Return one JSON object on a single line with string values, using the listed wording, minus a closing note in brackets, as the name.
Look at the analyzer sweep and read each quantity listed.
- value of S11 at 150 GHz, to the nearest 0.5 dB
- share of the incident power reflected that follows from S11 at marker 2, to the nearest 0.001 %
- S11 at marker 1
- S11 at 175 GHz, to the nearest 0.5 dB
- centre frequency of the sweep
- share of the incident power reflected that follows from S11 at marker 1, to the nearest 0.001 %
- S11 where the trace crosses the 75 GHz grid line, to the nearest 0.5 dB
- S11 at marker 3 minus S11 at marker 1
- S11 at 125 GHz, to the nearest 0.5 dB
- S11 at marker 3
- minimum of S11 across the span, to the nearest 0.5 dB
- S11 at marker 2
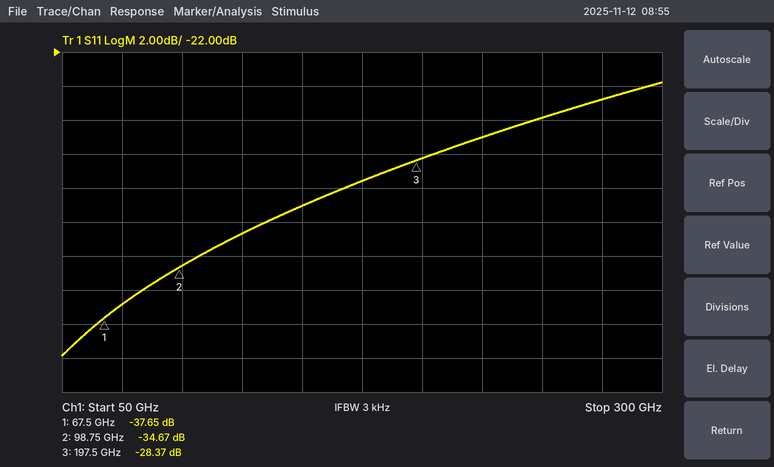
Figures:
{"value of S11 at 150 GHz, to the nearest 0.5 dB": "-31.0 dB", "share of the incident power reflected that follows from S11 at marker 2, to the nearest 0.001 %": "0.034 %", "S11 at marker 1": "-37.65 dB", "S11 at 175 GHz, to the nearest 0.5 dB": "-29.5 dB", "centre frequency of the sweep": "175 GHz", "share of the incident power reflected that follows from S11 at marker 1, to the nearest 0.001 %": "0.017 %", "S11 where the trace crosses the 75 GHz grid line, to the nearest 0.5 dB": "-37.0 dB", "S11 at marker 3 minus S11 at marker 1": "9.28 dB", "S11 at 125 GHz, to the nearest 0.5 dB": "-32.5 dB", "S11 at marker 3": "-28.37 dB", "minimum of S11 across the span, to the nearest 0.5 dB": "-40.0 dB", "S11 at marker 2": "-34.67 dB"}
